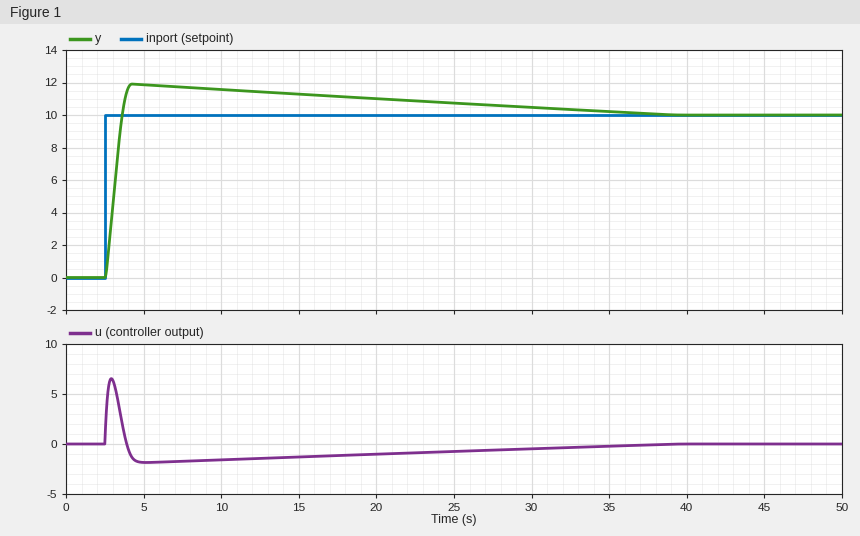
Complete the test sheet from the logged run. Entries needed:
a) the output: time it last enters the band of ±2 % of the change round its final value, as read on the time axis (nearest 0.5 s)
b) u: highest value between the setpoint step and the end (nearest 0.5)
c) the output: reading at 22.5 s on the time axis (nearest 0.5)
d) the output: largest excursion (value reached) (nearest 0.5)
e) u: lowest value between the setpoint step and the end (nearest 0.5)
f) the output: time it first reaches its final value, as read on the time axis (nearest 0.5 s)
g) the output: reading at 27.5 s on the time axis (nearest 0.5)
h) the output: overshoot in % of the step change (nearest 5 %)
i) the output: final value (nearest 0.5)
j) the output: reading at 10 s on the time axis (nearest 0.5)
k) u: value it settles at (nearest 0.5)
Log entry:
35.0 s
6.5
11.0
12.0
-2.0
3.5 s
10.5
20 %
10.0
11.5
0.0
